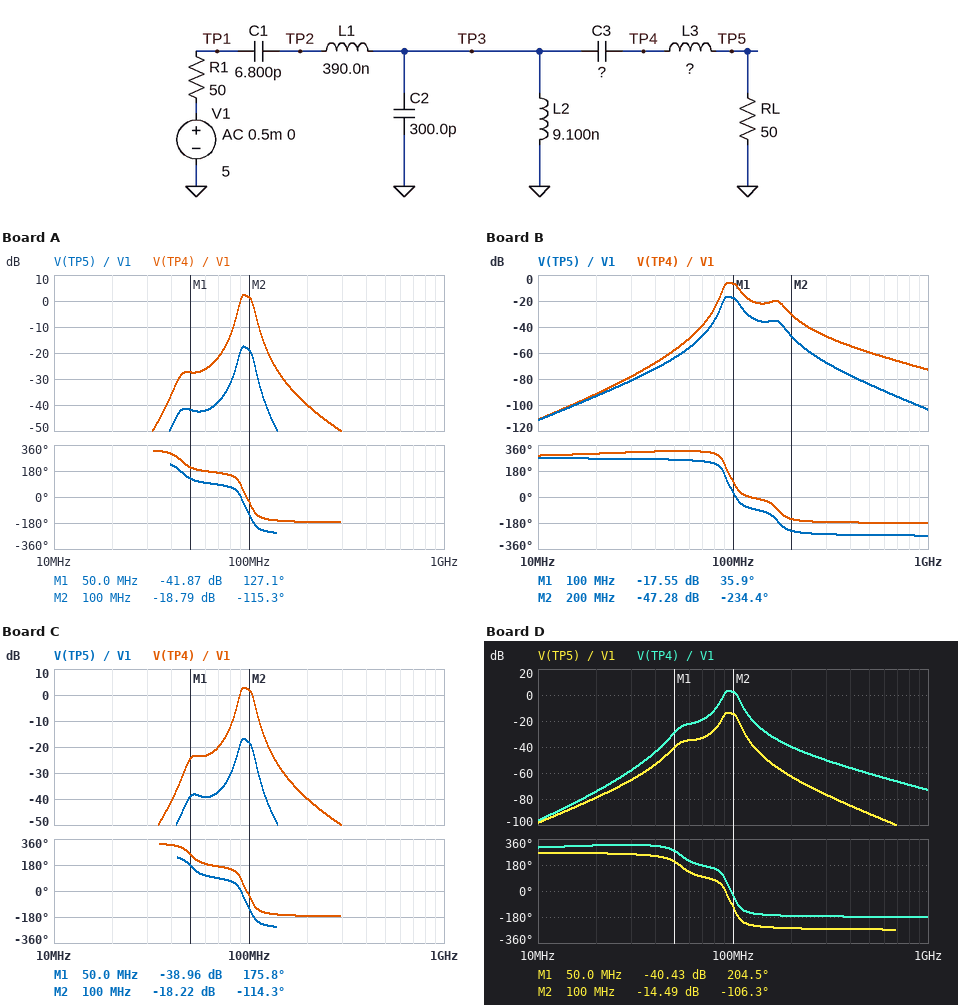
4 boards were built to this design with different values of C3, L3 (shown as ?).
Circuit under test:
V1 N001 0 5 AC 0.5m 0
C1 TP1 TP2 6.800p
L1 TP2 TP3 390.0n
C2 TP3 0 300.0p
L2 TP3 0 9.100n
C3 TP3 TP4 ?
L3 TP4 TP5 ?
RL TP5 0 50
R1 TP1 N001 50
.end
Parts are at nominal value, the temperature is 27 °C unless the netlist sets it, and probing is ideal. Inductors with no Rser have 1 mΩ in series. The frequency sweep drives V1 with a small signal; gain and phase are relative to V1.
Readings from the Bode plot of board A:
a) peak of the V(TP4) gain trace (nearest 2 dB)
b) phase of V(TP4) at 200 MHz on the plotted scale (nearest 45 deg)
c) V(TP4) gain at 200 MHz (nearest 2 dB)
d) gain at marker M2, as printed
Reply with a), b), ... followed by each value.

a) 2 dB
b) -180 deg
c) -40 dB
d) -18.79 dB
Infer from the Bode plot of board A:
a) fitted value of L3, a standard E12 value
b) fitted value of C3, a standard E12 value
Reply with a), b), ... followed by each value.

a) 820 nH
b) 15 pF
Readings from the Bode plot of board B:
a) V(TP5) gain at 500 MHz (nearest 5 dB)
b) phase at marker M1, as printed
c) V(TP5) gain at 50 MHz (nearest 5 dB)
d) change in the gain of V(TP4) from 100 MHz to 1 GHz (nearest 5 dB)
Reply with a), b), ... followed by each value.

a) -85 dB
b) 35.9 deg
c) -65 dB
d) -65 dB
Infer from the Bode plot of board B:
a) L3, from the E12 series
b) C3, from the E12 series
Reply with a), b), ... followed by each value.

a) 270 nH
b) 3.3 pF
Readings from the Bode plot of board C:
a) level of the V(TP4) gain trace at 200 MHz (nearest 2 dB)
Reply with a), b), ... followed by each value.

a) -40 dB
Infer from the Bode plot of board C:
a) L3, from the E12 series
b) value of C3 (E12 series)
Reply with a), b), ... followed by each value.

a) 820 nH
b) 12 pF
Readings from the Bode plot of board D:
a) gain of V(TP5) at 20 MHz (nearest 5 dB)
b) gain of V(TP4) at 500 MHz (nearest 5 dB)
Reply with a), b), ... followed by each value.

a) -80 dB
b) -60 dB
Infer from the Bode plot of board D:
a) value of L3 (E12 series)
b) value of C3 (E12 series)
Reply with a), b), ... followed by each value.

a) 560 nH
b) 15 pF
